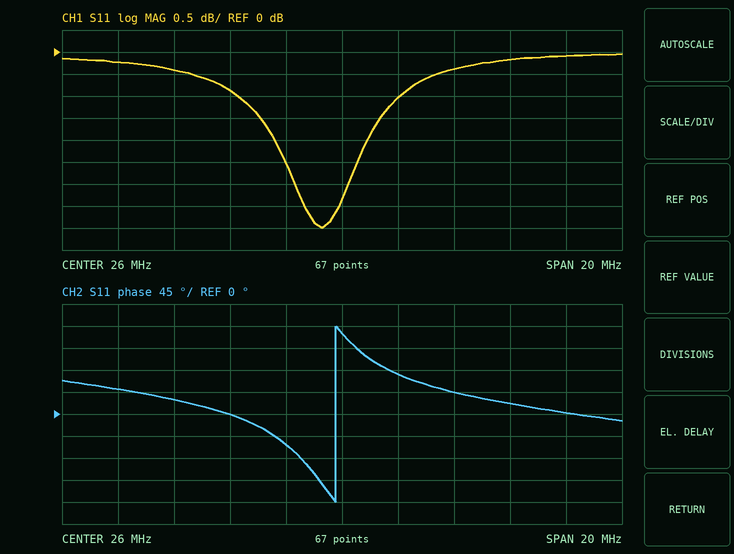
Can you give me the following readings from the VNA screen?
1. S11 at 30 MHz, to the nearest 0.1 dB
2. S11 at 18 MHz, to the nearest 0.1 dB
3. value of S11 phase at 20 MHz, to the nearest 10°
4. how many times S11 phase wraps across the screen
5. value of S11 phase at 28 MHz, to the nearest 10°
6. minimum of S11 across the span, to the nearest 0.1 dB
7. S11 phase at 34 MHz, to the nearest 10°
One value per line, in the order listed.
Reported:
-0.4 dB
-0.2 dB
30°
1
80°
-4.0 dB
0°
